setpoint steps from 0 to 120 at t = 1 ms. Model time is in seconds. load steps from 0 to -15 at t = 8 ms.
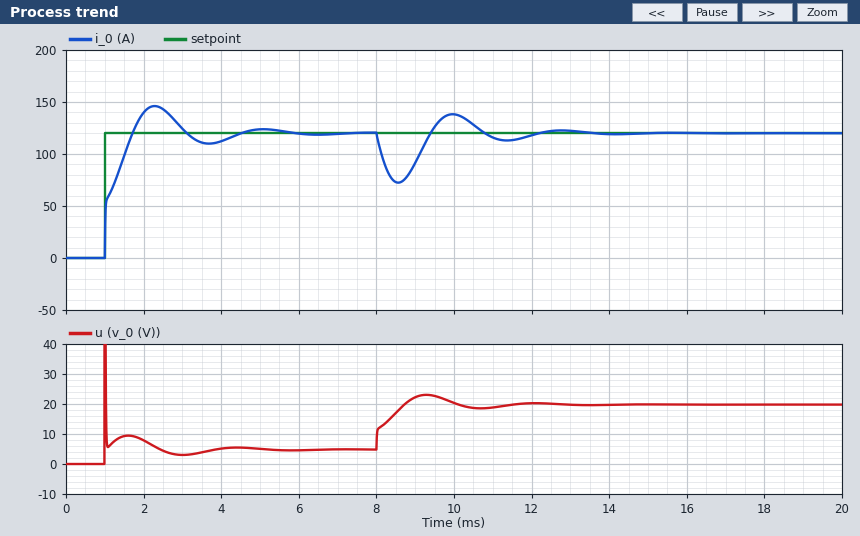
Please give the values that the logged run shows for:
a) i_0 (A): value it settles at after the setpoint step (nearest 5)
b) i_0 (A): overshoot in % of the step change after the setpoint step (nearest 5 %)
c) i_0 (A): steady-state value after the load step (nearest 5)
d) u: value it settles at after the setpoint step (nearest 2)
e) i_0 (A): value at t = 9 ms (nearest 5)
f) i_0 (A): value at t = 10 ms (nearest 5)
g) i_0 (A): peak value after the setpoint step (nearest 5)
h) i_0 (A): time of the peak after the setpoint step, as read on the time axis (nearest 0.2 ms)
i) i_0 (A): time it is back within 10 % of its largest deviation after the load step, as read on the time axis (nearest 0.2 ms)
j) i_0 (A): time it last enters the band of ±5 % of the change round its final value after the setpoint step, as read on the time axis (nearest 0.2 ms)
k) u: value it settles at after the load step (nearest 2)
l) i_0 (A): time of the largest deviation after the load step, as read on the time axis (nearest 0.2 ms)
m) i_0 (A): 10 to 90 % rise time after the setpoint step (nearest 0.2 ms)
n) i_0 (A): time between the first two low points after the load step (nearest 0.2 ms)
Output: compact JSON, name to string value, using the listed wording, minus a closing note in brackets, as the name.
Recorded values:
{"i_0 (A): value it settles at after the setpoint step": "120", "i_0 (A): overshoot in % of the step change after the setpoint step": "20 %", "i_0 (A): steady-state value after the load step": "120", "u: value it settles at after the setpoint step": "4", "i_0 (A): value at t = 9 ms": "90", "i_0 (A): value at t = 10 ms": "140", "i_0 (A): peak value after the setpoint step": "145", "i_0 (A): time of the peak after the setpoint step, as read on the time axis": "2.2 ms", "i_0 (A): time it is back within 10 % of its largest deviation after the load step, as read on the time axis": "11.8 ms", "i_0 (A): time it last enters the band of ±5 % of the change round its final value after the setpoint step, as read on the time axis": "4.2 ms", "u: value it settles at after the load step": "20", "i_0 (A): time of the largest deviation after the load step, as read on the time axis": "8.6 ms", "i_0 (A): 10 to 90 % rise time after the setpoint step": "0.6 ms", "i_0 (A): time between the first two low points after the load step": "2.8 ms"}
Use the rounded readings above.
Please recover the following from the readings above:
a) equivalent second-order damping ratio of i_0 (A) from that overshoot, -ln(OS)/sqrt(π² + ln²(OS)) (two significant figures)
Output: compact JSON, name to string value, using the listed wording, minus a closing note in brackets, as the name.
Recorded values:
{"equivalent second-order damping ratio of i_0 (A) from that overshoot, -ln(OS)/sqrt(π² + ln²(OS))": "0.46"}
